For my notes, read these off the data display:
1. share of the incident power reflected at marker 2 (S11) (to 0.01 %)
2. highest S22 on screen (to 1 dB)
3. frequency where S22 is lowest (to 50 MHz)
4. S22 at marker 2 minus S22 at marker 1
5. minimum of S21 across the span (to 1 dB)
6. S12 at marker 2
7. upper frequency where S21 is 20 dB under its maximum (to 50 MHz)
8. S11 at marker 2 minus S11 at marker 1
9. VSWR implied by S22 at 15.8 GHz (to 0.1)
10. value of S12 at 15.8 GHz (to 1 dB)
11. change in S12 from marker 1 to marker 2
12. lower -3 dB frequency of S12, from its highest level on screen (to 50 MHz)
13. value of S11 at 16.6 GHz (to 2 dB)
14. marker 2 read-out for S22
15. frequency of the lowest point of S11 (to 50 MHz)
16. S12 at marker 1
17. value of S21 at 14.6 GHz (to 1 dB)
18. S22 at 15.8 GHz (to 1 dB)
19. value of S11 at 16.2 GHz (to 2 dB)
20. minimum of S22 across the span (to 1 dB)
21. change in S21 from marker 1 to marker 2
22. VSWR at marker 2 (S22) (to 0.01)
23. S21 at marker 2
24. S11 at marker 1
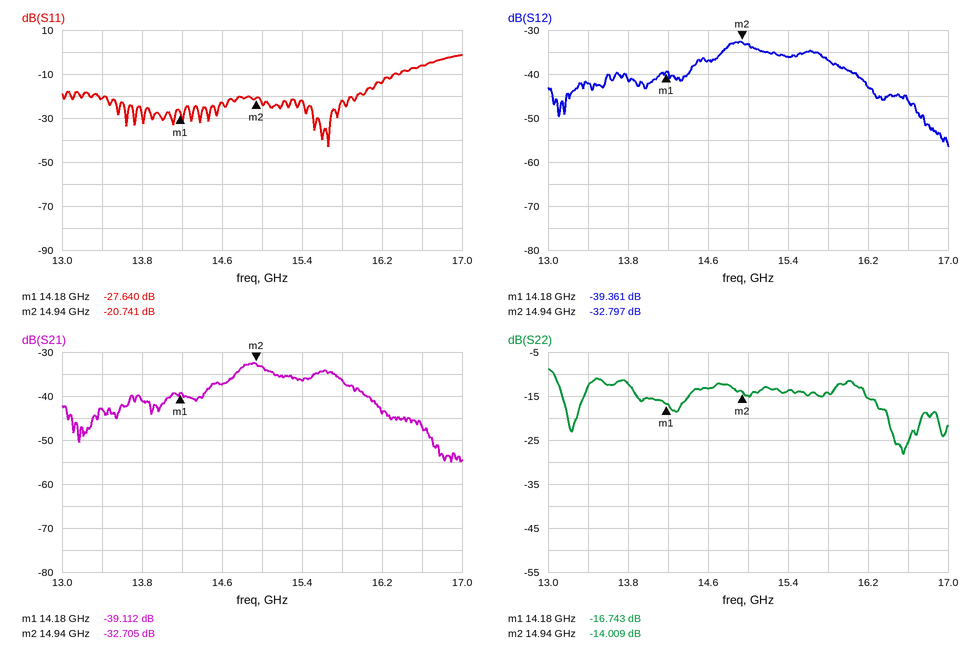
0.84 %
-9 dB
16.55 GHz
2.734 dB
-55 dB
-32.797 dB
16.75 GHz
6.899 dB
1.5
-37 dB
6.564 dB
14.70 GHz
-6 dB
-14.009 dB
15.65 GHz
-39.361 dB
-37 dB
-14 dB
-14 dB
-28 dB
6.407 dB
1.50
-32.705 dB
-27.640 dB
